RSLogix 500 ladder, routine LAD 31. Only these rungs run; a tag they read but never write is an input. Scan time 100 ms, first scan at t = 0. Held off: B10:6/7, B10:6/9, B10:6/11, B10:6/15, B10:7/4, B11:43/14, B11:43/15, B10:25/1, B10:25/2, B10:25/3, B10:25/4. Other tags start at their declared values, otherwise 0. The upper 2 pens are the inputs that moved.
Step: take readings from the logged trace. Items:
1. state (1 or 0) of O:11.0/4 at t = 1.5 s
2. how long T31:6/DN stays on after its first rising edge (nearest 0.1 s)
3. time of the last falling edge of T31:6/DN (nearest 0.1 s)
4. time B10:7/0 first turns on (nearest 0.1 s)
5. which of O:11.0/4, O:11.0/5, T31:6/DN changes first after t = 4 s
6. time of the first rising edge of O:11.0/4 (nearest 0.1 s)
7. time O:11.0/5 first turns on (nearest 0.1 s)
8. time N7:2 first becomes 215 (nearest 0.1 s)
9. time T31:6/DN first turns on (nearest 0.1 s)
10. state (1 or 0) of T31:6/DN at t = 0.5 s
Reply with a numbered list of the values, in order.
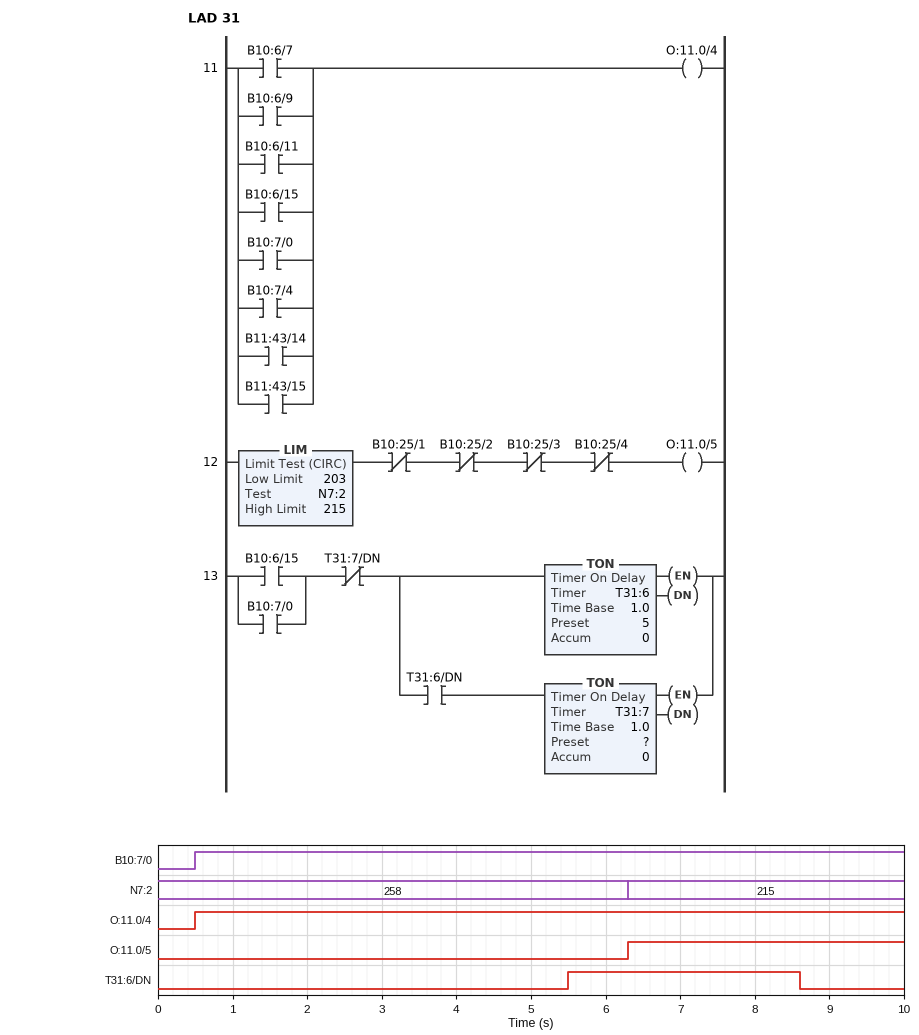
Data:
1. 1
2. 3.1 s
3. 8.6 s
4. 0.5 s
5. T31:6/DN
6. 0.5 s
7. 6.3 s
8. 6.3 s
9. 5.5 s
10. 0
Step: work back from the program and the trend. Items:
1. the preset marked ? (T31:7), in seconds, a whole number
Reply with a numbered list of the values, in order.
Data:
1. 3 s
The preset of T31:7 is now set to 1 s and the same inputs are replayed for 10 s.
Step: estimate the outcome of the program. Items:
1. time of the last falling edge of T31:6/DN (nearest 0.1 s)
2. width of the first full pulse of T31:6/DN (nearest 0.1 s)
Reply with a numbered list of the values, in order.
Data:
1. 6.6 s
2. 1.1 s
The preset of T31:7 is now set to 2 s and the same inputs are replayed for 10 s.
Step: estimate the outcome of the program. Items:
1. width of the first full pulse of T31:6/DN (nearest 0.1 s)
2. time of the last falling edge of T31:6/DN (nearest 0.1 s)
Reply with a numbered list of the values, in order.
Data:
1. 2.1 s
2. 7.6 s
